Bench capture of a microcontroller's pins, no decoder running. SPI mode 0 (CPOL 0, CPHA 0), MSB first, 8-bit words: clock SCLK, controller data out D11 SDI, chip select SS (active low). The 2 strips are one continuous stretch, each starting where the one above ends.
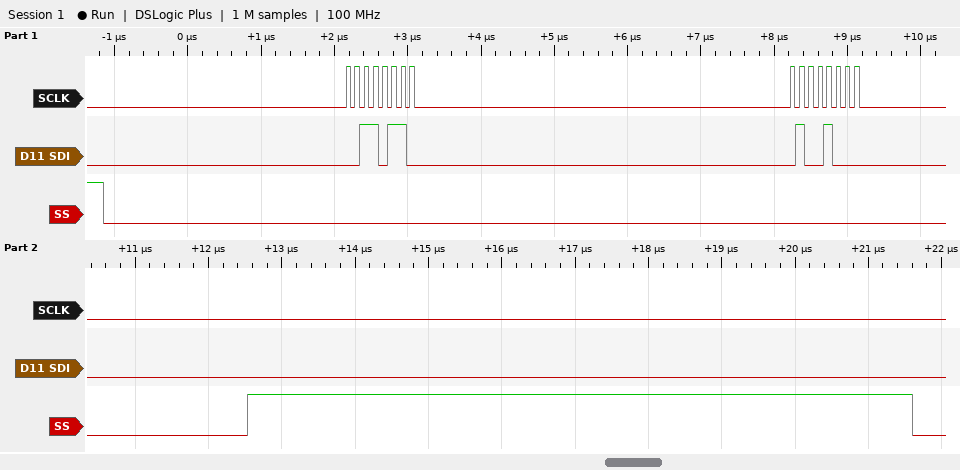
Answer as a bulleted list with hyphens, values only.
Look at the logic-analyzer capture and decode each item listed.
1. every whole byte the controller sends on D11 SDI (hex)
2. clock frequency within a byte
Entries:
- 36 48
- 8 MHz
